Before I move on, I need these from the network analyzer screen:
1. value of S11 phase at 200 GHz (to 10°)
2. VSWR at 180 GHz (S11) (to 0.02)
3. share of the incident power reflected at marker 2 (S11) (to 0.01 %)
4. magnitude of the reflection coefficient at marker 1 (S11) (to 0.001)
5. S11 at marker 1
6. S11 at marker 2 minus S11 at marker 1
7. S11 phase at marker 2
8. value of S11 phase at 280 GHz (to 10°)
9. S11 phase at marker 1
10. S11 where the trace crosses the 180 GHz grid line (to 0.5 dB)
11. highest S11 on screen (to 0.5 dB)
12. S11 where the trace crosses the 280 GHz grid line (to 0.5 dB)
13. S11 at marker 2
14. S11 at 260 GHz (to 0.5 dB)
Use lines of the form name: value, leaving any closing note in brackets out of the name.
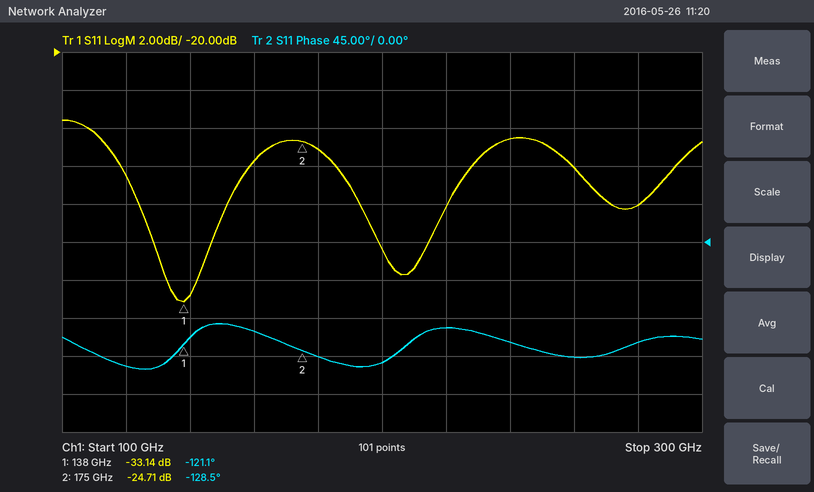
value of S11 phase at 200 GHz: -140°
VSWR at 180 GHz (S11): 1.12
share of the incident power reflected at marker 2 (S11): 0.34 %
magnitude of the reflection coefficient at marker 1 (S11): 0.022
S11 at marker 1: -33.14 dB
S11 at marker 2 minus S11 at marker 1: 8.43 dB
S11 phase at marker 2: -128.5°
value of S11 phase at 280 GHz: -120°
S11 phase at marker 1: -121.1°
S11 where the trace crosses the 180 GHz grid line: -25.0 dB
highest S11 on screen: -23.5 dB
S11 where the trace crosses the 280 GHz grid line: -28.0 dB
S11 at marker 2: -24.71 dB
S11 at 260 GHz: -26.0 dB
